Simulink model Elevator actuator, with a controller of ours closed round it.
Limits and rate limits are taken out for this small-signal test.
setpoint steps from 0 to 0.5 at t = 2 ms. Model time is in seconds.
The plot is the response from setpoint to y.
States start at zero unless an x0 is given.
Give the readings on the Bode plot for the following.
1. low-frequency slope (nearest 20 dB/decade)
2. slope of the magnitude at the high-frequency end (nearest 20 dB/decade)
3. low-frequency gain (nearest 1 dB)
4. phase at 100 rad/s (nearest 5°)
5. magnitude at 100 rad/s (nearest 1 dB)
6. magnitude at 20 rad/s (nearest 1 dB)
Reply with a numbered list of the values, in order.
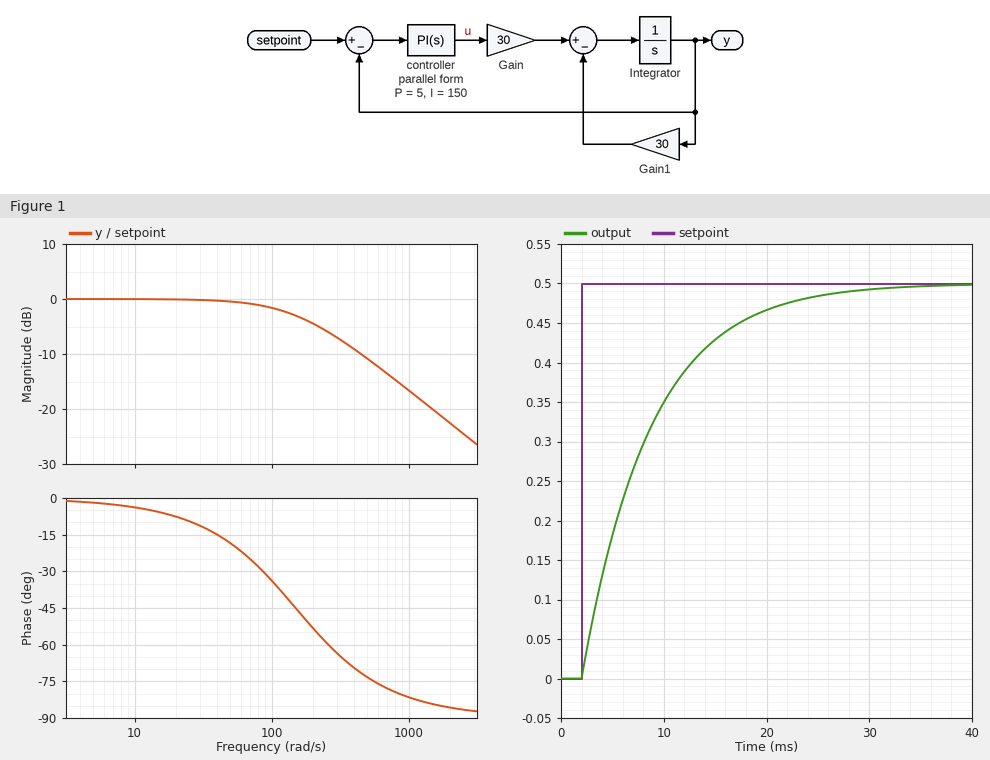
1. 0 dB/decade
2. -20 dB/decade
3. 0 dB
4. -35°
5. -2 dB
6. 0 dB
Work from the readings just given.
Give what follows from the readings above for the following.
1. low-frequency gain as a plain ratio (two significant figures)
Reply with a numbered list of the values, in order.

1. 1.0
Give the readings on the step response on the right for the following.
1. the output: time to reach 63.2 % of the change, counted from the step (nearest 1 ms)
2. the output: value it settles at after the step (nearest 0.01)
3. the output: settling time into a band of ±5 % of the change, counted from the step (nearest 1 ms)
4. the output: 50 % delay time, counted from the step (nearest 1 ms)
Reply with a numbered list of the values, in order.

1. 7 ms
2. 0.50
3. 20 ms
4. 5 ms
